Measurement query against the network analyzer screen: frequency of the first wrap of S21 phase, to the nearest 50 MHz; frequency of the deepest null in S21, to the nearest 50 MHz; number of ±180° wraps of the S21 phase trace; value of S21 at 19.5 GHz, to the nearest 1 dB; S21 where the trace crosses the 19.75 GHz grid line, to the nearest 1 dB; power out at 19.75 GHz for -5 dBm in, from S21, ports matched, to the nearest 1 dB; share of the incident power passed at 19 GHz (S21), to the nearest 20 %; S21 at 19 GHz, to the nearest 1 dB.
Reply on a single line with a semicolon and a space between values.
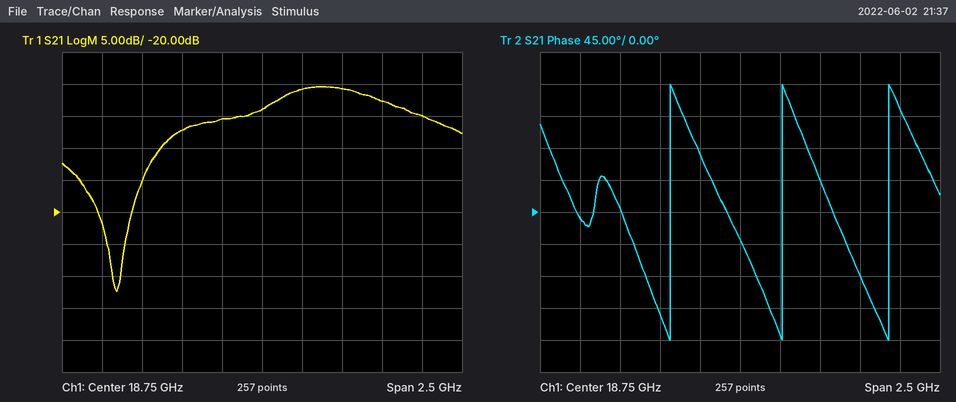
18.30 GHz; 17.85 GHz; 3; -3 dB; -5 dB; -10 dBm; 80 %; -1 dB
